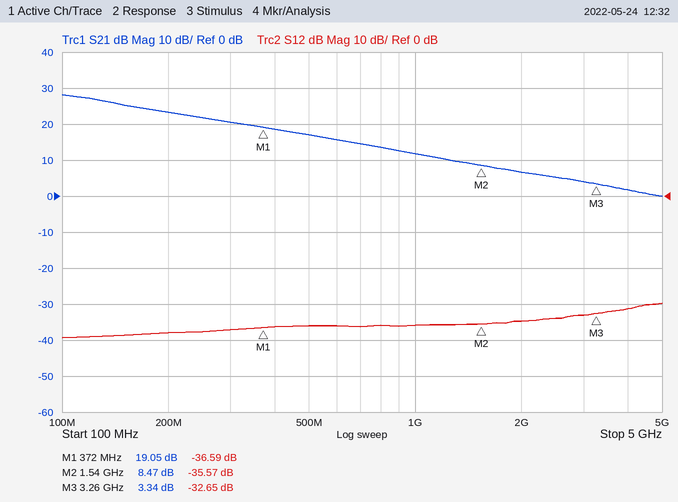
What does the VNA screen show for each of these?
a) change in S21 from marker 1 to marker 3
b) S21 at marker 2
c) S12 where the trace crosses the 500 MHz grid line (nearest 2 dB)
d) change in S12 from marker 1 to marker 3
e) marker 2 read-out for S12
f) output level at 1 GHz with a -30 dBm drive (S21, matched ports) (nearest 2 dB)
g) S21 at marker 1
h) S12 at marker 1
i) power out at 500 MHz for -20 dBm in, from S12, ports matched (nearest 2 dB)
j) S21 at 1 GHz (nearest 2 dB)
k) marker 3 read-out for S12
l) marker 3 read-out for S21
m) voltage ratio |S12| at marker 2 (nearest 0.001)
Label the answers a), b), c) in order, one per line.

a) -15.71 dB
b) 8.47 dB
c) -36 dB
d) 3.94 dB
e) -35.57 dB
f) -18 dBm
g) 19.05 dB
h) -36.59 dB
i) -56 dBm
j) 12 dB
k) -32.65 dB
l) 3.34 dB
m) 0.017
